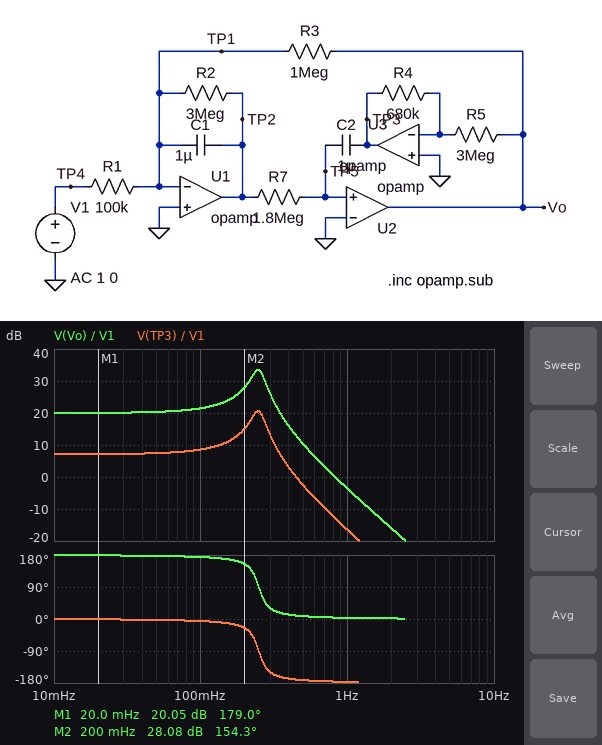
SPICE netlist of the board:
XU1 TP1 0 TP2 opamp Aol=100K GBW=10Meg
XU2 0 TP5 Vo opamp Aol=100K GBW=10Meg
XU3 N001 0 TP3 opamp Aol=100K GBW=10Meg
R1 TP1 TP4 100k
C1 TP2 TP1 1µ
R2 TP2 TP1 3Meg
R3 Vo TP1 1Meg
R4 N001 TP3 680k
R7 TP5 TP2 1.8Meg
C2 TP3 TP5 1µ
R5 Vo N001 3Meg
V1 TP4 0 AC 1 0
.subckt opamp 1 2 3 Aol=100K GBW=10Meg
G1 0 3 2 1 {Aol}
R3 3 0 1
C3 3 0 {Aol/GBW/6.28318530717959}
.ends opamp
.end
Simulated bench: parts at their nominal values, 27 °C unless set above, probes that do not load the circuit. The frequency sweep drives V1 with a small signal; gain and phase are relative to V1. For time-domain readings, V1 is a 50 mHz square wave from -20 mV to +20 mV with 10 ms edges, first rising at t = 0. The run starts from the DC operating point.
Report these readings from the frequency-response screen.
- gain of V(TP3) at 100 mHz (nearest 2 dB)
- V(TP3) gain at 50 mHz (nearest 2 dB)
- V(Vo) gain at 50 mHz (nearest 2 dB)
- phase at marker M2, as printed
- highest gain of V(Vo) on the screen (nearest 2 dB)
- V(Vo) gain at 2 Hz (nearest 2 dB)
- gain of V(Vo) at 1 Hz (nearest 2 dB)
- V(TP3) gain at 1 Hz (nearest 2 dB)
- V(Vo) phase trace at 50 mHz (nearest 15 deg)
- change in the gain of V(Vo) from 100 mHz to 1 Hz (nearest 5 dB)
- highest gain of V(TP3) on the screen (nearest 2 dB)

8 dB
8 dB
20 dB
154.3 deg
34 dB
-16 dB
-4 dB
-16 dB
180 deg
-25 dB
20 dB
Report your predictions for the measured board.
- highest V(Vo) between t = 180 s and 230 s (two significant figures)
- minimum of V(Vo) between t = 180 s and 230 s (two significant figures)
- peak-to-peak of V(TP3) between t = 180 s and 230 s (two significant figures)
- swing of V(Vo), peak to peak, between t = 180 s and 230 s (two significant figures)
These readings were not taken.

550 mV
-550 mV
250 mV
1.1 V
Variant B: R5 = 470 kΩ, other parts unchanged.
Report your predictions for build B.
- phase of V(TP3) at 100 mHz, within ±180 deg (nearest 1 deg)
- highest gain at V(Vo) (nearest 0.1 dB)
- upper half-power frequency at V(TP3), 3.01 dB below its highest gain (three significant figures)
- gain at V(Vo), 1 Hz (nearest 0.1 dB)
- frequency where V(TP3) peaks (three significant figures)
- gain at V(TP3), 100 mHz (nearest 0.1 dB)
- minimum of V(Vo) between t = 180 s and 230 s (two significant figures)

-93 deg
25.7 dB
116 mHz
-20.2 dB
91.2 mHz
28.5 dB
-340 mV
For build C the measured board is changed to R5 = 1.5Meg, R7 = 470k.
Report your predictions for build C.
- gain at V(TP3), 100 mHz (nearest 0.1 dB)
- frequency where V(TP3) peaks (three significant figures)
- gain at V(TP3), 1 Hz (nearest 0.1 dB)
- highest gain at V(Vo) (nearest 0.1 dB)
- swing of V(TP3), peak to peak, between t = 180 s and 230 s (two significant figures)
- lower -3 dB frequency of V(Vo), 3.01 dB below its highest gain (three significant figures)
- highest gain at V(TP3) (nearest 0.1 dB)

13.9 dB
343 mHz
-4.3 dB
36.3 dB
520 mV
315 mHz
29.4 dB
